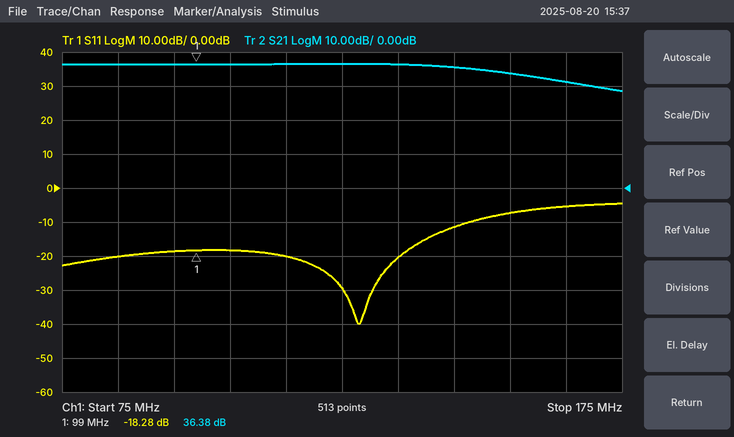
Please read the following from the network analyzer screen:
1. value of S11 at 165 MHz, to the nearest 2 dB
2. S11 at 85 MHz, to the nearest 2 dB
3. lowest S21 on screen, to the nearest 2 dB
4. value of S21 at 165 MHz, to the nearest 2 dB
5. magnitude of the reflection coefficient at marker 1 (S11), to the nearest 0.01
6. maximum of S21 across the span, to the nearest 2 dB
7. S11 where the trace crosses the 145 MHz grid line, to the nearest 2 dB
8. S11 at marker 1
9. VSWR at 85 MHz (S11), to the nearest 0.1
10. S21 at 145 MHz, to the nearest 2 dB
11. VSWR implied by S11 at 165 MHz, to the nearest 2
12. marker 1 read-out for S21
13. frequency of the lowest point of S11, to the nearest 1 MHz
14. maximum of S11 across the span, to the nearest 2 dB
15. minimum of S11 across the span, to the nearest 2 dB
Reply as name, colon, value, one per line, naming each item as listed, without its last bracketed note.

value of S11 at 165 MHz, to the nearest 2 dB: -6 dB
S11 at 85 MHz, to the nearest 2 dB: -20 dB
lowest S21 on screen, to the nearest 2 dB: 28 dB
value of S21 at 165 MHz, to the nearest 2 dB: 32 dB
magnitude of the reflection coefficient at marker 1 (S11), to the nearest 0.01: 0.12
maximum of S21 across the span, to the nearest 2 dB: 36 dB
S11 where the trace crosses the 145 MHz grid line, to the nearest 2 dB: -12 dB
S11 at marker 1: -18.28 dB
VSWR at 85 MHz (S11), to the nearest 0.1: 1.2
S21 at 145 MHz, to the nearest 2 dB: 36 dB
VSWR implied by S11 at 165 MHz, to the nearest 2: 4
marker 1 read-out for S21: 36.38 dB
frequency of the lowest point of S11, to the nearest 1 MHz: 128 MHz
maximum of S11 across the span, to the nearest 2 dB: -4 dB
minimum of S11 across the span, to the nearest 2 dB: -40 dB
